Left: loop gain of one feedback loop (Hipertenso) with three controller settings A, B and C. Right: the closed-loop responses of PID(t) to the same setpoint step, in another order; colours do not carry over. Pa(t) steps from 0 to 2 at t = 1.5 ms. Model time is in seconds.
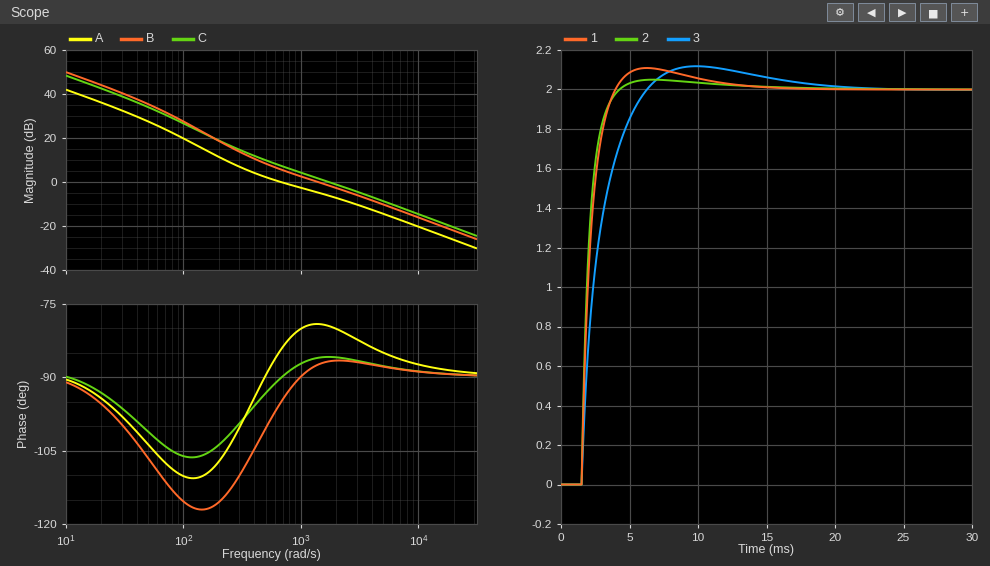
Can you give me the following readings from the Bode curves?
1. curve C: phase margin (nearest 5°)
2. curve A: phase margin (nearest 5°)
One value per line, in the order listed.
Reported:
95°
95°
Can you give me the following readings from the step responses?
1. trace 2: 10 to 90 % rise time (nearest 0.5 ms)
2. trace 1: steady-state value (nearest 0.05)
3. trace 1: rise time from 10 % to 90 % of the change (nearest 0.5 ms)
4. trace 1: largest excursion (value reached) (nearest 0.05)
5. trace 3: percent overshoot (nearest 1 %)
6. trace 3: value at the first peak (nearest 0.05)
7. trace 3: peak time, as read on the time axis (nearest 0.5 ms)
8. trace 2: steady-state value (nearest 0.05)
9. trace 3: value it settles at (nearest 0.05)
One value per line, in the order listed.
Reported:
1.5 ms
2.00
1.5 ms
2.10
6 %
2.10
10.0 ms
2.00
2.00
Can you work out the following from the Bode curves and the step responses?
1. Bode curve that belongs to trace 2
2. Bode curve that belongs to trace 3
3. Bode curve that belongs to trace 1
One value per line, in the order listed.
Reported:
C
A
B
